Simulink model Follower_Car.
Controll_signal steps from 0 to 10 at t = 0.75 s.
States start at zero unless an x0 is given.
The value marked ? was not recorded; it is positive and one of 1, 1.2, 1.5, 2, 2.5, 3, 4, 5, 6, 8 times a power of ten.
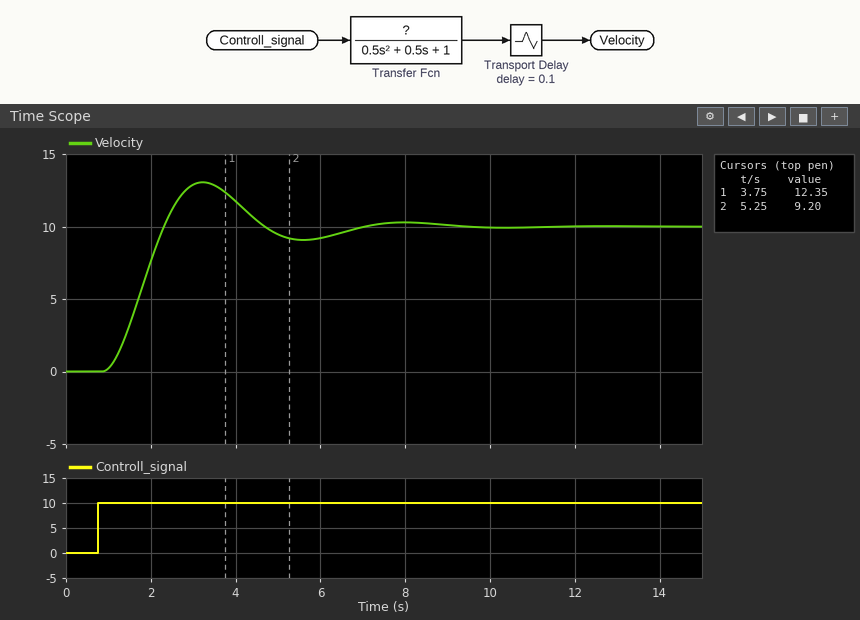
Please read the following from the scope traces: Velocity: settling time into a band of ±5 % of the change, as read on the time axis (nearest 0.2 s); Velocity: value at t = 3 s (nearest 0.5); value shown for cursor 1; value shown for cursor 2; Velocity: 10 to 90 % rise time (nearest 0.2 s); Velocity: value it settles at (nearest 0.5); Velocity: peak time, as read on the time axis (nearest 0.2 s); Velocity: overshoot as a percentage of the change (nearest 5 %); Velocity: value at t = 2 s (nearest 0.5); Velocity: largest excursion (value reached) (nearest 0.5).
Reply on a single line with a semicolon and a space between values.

6.4 s; 13.0; 12.35; 9.20; 1.0 s; 10.0; 3.2 s; 30 %; 7.5; 13.0
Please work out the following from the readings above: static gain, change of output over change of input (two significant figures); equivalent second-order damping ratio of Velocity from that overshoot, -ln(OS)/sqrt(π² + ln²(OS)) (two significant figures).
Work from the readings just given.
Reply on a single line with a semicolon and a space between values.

1.0; 0.36
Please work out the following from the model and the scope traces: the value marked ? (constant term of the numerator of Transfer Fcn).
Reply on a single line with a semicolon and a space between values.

1
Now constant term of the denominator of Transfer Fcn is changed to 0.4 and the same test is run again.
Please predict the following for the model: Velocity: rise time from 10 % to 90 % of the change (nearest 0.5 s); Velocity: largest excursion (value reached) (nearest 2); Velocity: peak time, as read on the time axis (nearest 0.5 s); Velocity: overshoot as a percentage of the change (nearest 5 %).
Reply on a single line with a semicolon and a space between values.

2.0 s; 28; 5.0 s; 10 %
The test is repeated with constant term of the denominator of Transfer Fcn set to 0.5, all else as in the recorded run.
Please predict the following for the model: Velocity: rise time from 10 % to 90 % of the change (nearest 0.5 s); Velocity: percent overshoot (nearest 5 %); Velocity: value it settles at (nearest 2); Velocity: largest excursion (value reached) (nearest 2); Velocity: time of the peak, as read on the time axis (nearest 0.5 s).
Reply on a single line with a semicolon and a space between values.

1.5 s; 15 %; 20; 24; 4.5 s
